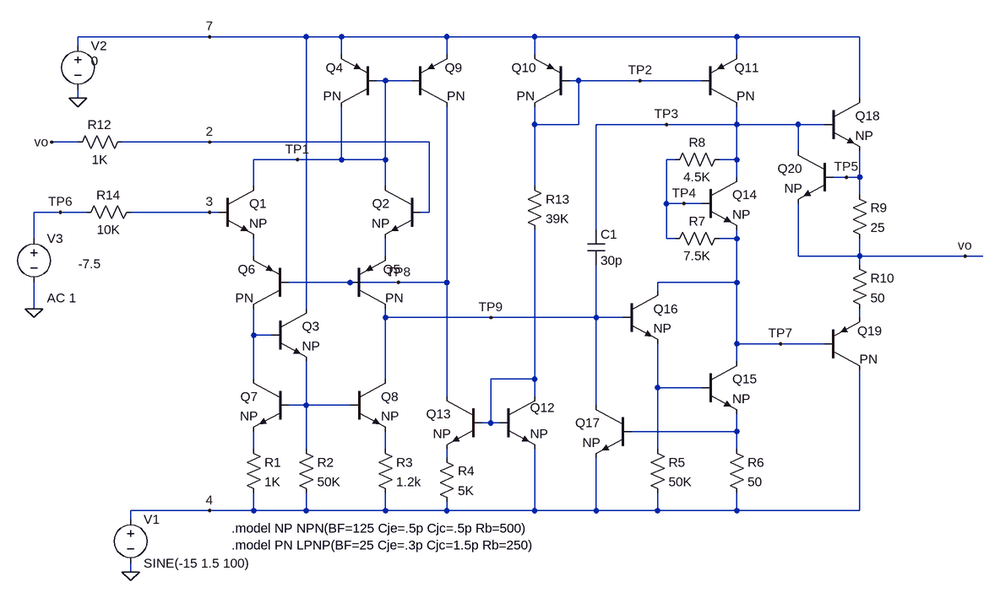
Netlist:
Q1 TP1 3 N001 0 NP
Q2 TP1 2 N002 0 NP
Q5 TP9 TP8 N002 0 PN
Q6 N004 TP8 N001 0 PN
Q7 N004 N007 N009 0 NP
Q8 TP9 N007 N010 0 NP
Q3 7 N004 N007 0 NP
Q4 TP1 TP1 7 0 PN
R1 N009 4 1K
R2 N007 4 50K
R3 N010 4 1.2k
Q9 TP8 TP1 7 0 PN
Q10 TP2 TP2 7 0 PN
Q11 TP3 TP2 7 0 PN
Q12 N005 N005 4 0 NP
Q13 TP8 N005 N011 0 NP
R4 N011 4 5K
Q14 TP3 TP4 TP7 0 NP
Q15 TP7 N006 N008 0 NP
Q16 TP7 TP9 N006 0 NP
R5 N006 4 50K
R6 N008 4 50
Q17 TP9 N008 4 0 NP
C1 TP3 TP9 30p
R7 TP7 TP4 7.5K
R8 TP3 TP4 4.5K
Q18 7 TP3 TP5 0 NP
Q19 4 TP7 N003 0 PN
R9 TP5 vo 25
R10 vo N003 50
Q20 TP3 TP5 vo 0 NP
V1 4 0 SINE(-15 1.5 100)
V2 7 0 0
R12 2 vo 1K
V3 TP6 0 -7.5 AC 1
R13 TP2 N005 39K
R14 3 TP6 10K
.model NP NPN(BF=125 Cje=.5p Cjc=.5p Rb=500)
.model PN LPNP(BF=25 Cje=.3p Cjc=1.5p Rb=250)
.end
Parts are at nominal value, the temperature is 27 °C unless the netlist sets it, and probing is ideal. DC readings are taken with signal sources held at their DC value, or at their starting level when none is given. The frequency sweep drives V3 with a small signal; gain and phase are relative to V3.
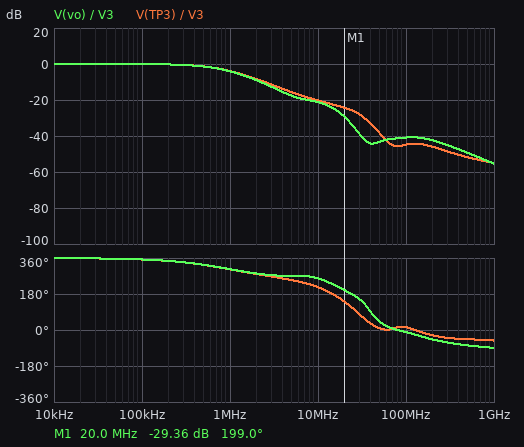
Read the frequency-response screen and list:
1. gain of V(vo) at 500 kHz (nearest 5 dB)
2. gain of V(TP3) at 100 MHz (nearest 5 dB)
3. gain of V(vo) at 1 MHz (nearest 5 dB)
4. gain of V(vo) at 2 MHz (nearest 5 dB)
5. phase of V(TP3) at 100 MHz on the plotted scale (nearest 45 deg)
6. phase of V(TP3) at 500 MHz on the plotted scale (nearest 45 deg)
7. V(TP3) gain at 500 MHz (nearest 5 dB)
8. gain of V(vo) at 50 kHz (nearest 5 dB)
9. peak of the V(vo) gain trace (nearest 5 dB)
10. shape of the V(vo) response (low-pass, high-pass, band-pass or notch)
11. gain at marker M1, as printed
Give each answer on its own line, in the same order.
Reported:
0 dB
-45 dB
-5 dB
-10 dB
0 deg
-45 deg
-50 dB
0 dB
0 dB
low-pass
-29.36 dB
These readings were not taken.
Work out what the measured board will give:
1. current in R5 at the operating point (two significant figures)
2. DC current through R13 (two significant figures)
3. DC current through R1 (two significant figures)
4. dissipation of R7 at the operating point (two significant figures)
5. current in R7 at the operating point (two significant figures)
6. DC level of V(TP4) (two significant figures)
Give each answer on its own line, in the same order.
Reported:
15 µA
350 µA
8.2 µA
72 µW
98 µA
-7.4 V
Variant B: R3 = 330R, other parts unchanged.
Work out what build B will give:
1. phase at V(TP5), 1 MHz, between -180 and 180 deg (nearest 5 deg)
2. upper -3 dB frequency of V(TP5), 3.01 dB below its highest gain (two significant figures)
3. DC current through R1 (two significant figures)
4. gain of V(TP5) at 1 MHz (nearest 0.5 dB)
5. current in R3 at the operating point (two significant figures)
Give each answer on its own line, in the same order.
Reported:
-50 deg
1.0 MHz
7.3 µA
-3.0 dB
8.7 µA
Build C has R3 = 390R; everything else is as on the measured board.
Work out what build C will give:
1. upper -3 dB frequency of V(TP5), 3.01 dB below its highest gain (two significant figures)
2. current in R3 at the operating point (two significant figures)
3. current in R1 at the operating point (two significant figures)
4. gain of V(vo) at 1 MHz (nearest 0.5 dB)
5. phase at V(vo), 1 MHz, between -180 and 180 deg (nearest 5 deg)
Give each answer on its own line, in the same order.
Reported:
1.0 MHz
8.6 µA
7.4 µA
-3.0 dB
-50 deg
